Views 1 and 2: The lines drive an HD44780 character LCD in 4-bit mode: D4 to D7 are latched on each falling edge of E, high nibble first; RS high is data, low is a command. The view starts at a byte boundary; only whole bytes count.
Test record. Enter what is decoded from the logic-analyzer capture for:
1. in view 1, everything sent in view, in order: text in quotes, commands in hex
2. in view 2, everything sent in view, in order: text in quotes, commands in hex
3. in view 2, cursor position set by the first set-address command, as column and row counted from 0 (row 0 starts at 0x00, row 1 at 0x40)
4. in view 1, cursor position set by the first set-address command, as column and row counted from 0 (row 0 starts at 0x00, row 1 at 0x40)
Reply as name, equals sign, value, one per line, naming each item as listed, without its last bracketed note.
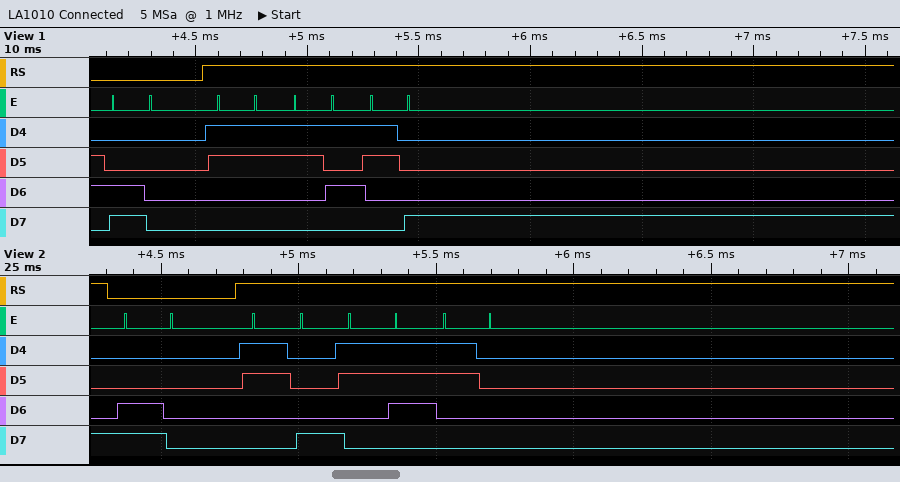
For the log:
in view 1, everything sent in view, in order: text in quotes, commands in hex = 0xC0 "358"
in view 2, everything sent in view, in order: text in quotes, commands in hex = 0xC0 "870"
in view 2, cursor position set by the first set-address command, as column and row counted from 0 = column 0, row 1
in view 1, cursor position set by the first set-address command, as column and row counted from 0 = column 0, row 1
